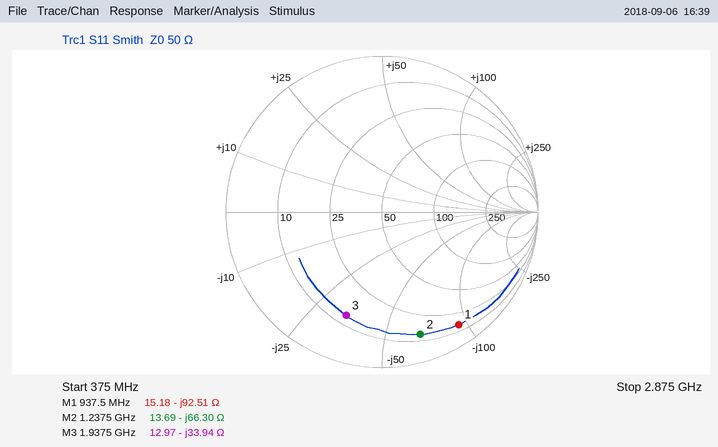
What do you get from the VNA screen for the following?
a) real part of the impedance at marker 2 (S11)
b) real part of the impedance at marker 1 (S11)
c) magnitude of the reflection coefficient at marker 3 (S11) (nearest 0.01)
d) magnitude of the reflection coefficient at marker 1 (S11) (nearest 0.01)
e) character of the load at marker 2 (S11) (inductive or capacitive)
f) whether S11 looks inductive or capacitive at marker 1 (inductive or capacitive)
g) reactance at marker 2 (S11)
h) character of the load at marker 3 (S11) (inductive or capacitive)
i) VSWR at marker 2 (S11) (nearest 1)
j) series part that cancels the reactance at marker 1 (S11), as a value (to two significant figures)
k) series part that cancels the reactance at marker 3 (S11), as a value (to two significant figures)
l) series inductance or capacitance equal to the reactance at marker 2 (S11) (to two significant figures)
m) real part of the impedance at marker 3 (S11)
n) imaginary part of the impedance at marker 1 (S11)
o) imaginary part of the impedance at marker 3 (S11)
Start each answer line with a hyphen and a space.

- 13.69 Ω
- 15.18 Ω
- 0.70
- 0.87
- capacitive
- capacitive
- -66.30 Ω
- capacitive
- 10
- 16 nH
- 2.8 nH
- 1.9 pF
- 12.97 Ω
- -92.51 Ω
- -33.94 Ω
